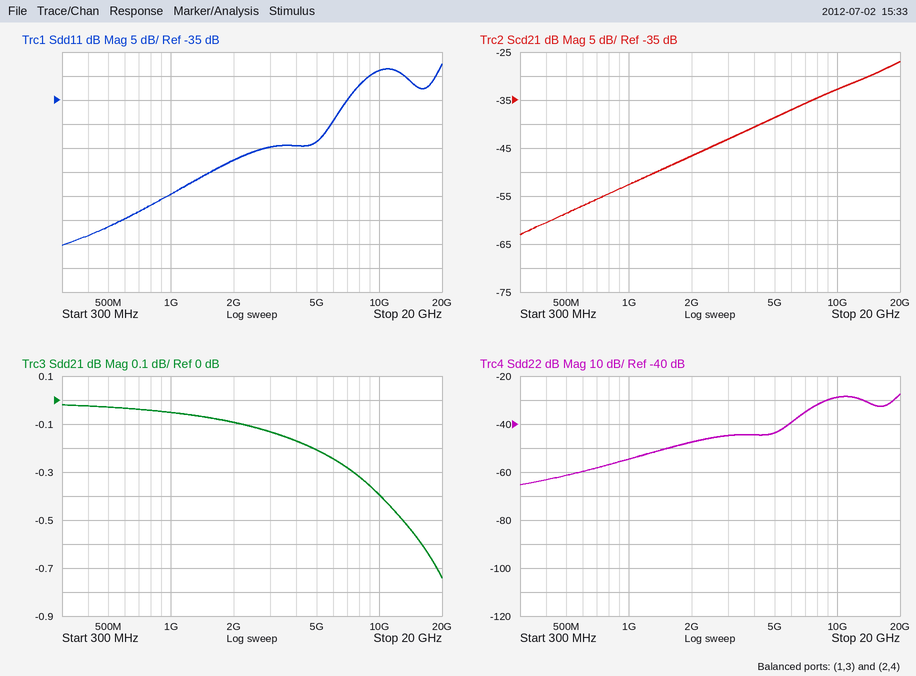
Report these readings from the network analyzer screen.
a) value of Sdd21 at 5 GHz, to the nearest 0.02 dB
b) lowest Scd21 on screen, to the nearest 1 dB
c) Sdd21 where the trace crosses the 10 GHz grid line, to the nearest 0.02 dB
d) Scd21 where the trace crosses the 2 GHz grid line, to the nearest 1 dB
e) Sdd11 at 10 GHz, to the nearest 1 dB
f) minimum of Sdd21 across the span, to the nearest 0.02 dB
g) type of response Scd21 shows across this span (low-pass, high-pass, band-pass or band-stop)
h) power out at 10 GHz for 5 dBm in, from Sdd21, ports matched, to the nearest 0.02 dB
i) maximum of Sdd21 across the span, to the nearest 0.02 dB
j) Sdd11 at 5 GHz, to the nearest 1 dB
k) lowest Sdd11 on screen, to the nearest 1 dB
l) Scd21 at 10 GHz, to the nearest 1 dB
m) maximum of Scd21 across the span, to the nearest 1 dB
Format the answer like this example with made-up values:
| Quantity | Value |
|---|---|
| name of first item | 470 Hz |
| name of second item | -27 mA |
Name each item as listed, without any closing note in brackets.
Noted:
| Quantity | Value |
|---|---|
| value of Sdd21 at 5 GHz, to the nearest 0.02 dB | -0.20 dB |
| lowest Scd21 on screen, to the nearest 1 dB | -63 dB |
| Sdd21 where the trace crosses the 10 GHz grid line, to the nearest 0.02 dB | -0.40 dB |
| Scd21 where the trace crosses the 2 GHz grid line, to the nearest 1 dB | -47 dB |
| Sdd11 at 10 GHz, to the nearest 1 dB | -29 dB |
| minimum of Sdd21 across the span, to the nearest 0.02 dB | -0.74 dB |
| type of response Scd21 shows across this span | high-pass |
| power out at 10 GHz for 5 dBm in, from Sdd21, ports matched, to the nearest 0.02 dB | 4.60 dBm |
| maximum of Sdd21 across the span, to the nearest 0.02 dB | -0.02 dB |
| Sdd11 at 5 GHz, to the nearest 1 dB | -44 dB |
| lowest Sdd11 on screen, to the nearest 1 dB | -65 dB |
| Scd21 at 10 GHz, to the nearest 1 dB | -33 dB |
| maximum of Scd21 across the span, to the nearest 1 dB | -27 dB |
